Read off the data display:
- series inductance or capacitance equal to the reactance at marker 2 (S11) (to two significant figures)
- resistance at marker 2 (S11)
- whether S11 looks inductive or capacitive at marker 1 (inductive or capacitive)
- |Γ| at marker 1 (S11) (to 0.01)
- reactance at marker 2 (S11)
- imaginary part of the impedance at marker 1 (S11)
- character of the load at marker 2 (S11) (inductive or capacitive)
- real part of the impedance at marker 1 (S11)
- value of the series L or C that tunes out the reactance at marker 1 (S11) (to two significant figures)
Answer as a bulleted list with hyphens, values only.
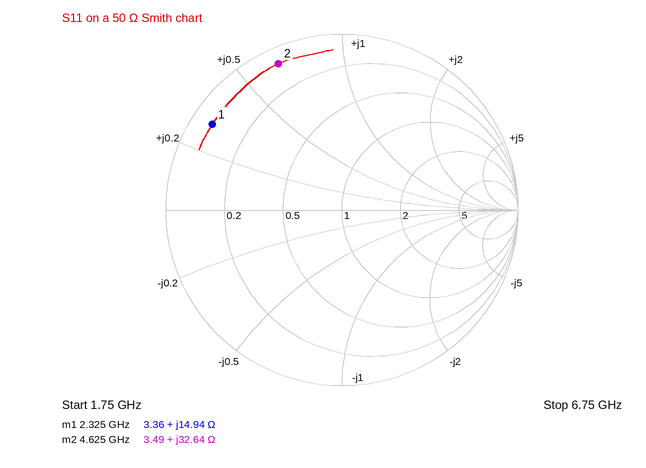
- 1.1 nH
- 3.49 Ω
- inductive
- 0.88
- +32.64 Ω
- +14.94 Ω
- inductive
- 3.36 Ω
- 4.6 pF
